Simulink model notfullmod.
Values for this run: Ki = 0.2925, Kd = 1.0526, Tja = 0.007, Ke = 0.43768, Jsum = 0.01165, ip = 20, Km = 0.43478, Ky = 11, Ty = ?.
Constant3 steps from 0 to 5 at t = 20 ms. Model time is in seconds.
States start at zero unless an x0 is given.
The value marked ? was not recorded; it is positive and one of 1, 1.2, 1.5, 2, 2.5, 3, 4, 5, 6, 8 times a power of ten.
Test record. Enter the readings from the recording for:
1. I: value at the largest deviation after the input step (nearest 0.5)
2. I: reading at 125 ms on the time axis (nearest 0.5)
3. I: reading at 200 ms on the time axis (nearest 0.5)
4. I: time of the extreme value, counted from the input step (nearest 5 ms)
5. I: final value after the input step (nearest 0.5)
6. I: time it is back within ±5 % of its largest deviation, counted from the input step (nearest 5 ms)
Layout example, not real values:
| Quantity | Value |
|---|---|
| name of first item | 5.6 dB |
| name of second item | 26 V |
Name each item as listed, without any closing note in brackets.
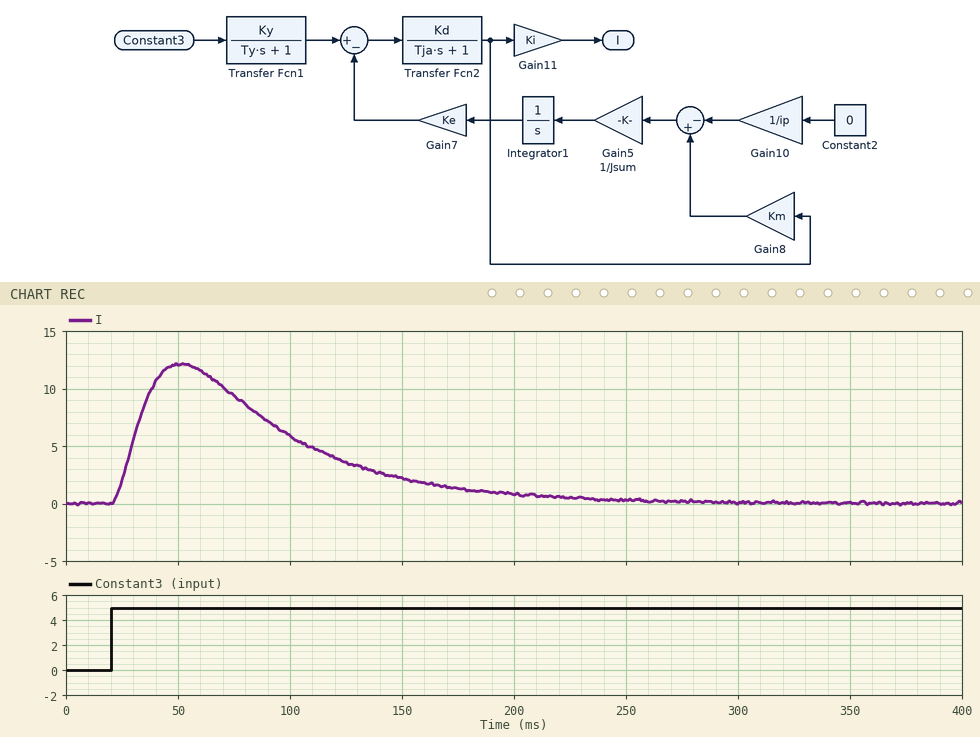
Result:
| Quantity | Value |
|---|---|
| I: value at the largest deviation after the input step | 12.0 |
| I: reading at 125 ms on the time axis | 3.5 |
| I: reading at 200 ms on the time axis | 1.0 |
| I: time of the extreme value, counted from the input step | 30 ms |
| I: final value after the input step | 0.0 |
| I: time it is back within ±5 % of its largest deviation, counted from the input step | 195 ms |
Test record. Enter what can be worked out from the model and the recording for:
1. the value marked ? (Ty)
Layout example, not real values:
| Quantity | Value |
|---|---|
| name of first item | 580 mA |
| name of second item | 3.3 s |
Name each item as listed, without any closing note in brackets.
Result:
| Quantity | Value |
|---|---|
| the value marked ? | 0.01 |
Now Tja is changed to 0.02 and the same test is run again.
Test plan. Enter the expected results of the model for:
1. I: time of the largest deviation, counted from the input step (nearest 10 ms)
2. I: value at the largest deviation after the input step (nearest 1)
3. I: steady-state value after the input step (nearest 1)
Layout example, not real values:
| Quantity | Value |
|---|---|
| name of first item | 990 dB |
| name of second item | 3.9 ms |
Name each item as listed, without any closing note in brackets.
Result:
| Quantity | Value |
|---|---|
| I: time of the largest deviation, counted from the input step | 50 ms |
| I: value at the largest deviation after the input step | 11 |
| I: steady-state value after the input step | 0 |
